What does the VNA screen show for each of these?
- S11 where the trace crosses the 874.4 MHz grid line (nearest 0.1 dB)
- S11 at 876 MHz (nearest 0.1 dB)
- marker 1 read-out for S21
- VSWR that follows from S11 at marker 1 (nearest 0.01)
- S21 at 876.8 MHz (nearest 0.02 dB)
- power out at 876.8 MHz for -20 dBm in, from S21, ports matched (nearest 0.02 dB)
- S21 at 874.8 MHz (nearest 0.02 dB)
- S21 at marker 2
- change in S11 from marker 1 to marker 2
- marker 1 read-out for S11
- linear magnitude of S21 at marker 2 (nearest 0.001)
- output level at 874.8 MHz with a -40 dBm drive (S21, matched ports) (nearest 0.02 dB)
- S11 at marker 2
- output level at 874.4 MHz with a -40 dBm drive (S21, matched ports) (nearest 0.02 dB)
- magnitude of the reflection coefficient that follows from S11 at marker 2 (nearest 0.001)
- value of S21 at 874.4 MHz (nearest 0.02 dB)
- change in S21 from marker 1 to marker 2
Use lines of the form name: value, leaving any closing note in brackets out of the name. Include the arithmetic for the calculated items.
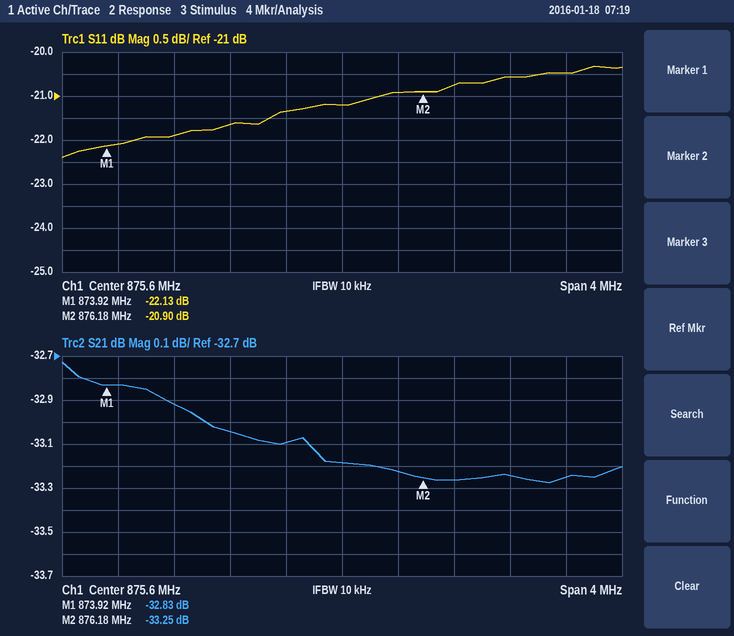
S11 where the trace crosses the 874.4 MHz grid line: -21.9 dB
S11 at 876 MHz: -20.9 dB
marker 1 read-out for S21: -32.83 dB
VSWR that follows from S11 at marker 1: (1 + 0.0783)/(1 − 0.0783) ≈ 1.17
S21 at 876.8 MHz: -33.24 dB
power out at 876.8 MHz for -20 dBm in, from S21, ports matched: -20 dBm + (-33.24 dB) = -53.24 dBm
S21 at 874.8 MHz: -33.04 dB
S21 at marker 2: -33.25 dB
change in S11 from marker 1 to marker 2: -20.9 − (-22.13) = 1.23 dB
marker 1 read-out for S11: -22.13 dB
linear magnitude of S21 at marker 2: 10^(-33.25/20) ≈ 0.022
output level at 874.8 MHz with a -40 dBm drive (S21, matched ports): -40 dBm + (-33.04 dB) = -73.04 dBm
S11 at marker 2: -20.90 dB
output level at 874.4 MHz with a -40 dBm drive (S21, matched ports): -40 dBm + (-32.92 dB) = -72.92 dBm
magnitude of the reflection coefficient that follows from S11 at marker 2: 10^(-20.9/20) ≈ 0.090
value of S21 at 874.4 MHz: -32.92 dB
change in S21 from marker 1 to marker 2: -33.25 − (-32.83) = -0.42 dB
